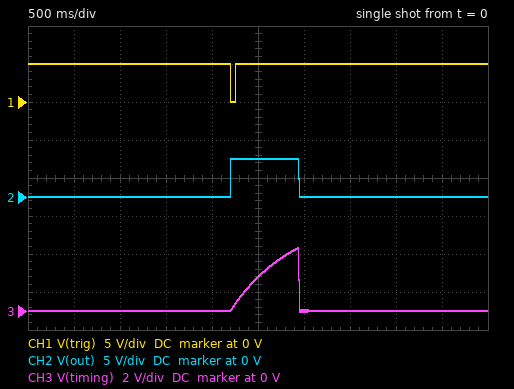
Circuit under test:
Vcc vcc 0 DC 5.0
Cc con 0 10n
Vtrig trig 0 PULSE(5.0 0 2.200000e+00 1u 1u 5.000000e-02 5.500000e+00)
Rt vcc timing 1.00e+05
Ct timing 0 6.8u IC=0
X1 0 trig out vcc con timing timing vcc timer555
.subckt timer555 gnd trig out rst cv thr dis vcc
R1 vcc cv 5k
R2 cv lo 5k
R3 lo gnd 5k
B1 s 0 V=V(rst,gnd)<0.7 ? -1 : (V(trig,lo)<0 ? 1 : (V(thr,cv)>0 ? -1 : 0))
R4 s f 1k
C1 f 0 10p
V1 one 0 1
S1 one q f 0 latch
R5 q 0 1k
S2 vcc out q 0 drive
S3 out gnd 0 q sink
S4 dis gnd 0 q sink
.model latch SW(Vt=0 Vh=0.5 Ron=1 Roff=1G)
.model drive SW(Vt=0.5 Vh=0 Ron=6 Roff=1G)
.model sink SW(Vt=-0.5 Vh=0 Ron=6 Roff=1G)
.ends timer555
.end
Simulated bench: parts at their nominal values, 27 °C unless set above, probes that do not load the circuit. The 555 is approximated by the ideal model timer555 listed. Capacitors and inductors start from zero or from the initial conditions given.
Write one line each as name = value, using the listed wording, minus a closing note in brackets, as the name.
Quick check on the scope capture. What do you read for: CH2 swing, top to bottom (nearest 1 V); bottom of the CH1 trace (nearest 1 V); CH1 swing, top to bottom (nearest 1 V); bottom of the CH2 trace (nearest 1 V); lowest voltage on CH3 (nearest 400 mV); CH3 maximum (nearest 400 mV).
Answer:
CH2 swing, top to bottom = 5 V
bottom of the CH1 trace = 0 V
CH1 swing, top to bottom = 5 V
bottom of the CH2 trace = 0 V
lowest voltage on CH3 = 0 V
CH3 maximum = 3.2 V
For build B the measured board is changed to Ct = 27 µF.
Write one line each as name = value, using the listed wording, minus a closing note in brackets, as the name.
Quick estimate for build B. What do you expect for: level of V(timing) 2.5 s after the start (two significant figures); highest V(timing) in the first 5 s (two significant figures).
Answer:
level of V(timing) 2.5 s after the start = 530 mV
highest V(timing) in the first 5 s = 3.2 V
